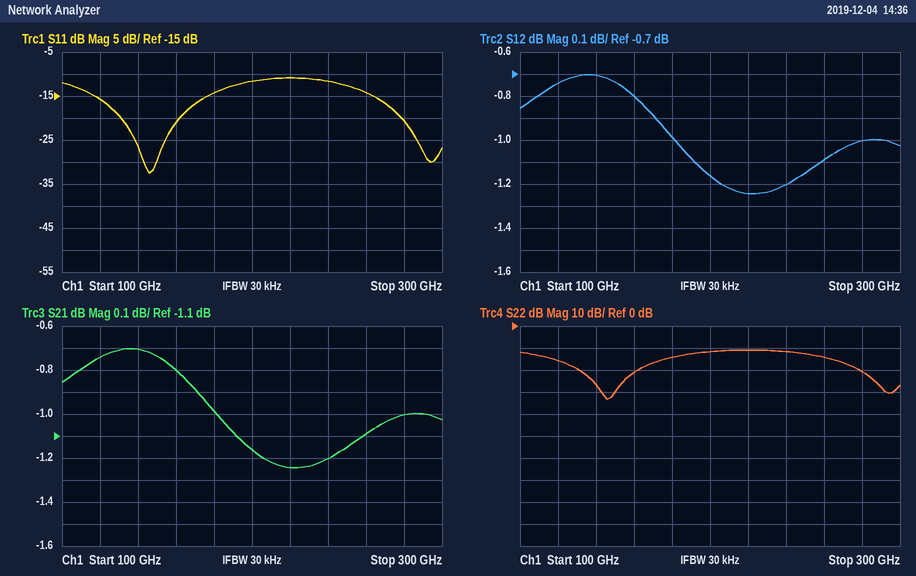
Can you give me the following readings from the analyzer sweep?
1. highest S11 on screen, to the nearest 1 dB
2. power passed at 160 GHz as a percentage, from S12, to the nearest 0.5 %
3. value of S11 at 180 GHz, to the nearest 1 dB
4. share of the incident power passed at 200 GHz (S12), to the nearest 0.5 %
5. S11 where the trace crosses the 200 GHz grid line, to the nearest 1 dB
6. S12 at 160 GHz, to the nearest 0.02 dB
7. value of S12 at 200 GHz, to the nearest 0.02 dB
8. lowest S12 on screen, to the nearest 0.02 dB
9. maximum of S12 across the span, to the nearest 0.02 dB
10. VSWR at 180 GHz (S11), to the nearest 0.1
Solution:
-11 dB
83.0 %
-14 dB
76.5 %
-12 dB
-0.80 dB
-1.16 dB
-1.24 dB
-0.70 dB
1.5
